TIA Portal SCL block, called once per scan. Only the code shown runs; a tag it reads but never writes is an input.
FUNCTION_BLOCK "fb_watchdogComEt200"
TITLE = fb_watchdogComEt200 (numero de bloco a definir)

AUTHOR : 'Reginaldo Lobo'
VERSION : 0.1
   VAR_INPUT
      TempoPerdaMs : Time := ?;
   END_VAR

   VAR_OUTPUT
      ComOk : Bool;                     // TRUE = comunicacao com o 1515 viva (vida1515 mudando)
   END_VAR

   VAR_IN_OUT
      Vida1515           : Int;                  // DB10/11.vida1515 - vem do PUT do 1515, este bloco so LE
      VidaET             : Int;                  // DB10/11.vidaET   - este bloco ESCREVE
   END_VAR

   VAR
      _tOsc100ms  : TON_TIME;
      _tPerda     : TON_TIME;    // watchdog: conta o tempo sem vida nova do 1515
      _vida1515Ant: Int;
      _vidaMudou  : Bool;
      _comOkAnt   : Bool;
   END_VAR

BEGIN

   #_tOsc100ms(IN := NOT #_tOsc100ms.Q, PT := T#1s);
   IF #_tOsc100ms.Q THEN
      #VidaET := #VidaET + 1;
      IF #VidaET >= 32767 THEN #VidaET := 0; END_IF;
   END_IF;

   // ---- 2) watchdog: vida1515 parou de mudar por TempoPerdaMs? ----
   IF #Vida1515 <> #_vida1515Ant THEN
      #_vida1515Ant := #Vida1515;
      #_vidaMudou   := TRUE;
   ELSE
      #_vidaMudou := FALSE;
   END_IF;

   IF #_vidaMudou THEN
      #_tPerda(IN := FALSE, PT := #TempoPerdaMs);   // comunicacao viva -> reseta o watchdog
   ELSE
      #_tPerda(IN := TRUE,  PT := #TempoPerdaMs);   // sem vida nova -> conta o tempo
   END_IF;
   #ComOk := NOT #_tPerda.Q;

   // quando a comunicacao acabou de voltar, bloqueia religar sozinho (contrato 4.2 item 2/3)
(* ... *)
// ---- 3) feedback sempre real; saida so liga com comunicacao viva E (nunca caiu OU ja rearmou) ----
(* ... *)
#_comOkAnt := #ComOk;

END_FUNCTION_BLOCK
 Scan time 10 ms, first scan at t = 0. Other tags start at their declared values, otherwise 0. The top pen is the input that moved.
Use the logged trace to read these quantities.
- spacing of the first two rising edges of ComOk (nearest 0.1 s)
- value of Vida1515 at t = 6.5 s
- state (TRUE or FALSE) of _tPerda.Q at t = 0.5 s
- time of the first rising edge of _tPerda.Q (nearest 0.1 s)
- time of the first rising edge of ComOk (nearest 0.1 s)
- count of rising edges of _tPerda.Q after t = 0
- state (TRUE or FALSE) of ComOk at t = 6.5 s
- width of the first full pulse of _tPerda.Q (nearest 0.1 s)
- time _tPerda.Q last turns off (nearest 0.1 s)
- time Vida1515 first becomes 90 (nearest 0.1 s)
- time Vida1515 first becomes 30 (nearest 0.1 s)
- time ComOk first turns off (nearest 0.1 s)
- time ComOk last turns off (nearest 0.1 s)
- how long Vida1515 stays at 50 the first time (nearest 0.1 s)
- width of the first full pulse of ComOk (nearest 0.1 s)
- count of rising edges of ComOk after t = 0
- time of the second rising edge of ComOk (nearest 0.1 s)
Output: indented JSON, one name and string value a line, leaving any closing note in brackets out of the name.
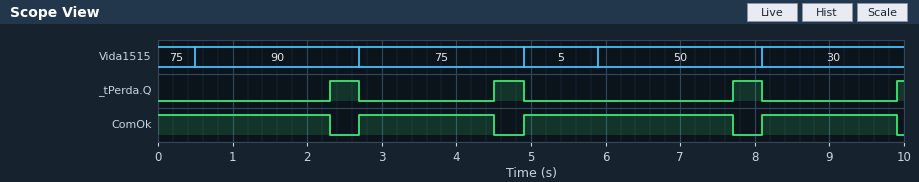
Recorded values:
{
  "spacing of the first two rising edges of ComOk": "2.2 s",
  "value of Vida1515 at t = 6.5 s": "50",
  "state (TRUE or FALSE) of _tPerda.Q at t = 0.5 s": "FALSE",
  "time of the first rising edge of _tPerda.Q": "2.3 s",
  "time of the first rising edge of ComOk": "2.7 s",
  "count of rising edges of _tPerda.Q after t = 0": "4",
  "state (TRUE or FALSE) of ComOk at t = 6.5 s": "TRUE",
  "width of the first full pulse of _tPerda.Q": "0.4 s",
  "time _tPerda.Q last turns off": "8.1 s",
  "time Vida1515 first becomes 90": "0.5 s",
  "time Vida1515 first becomes 30": "8.1 s",
  "time ComOk first turns off": "2.3 s",
  "time ComOk last turns off": "9.9 s",
  "how long Vida1515 stays at 50 the first time": "2.2 s",
  "width of the first full pulse of ComOk": "1.8 s",
  "count of rising edges of ComOk after t = 0": "3",
  "time of the second rising edge of ComOk": "4.9 s"
}
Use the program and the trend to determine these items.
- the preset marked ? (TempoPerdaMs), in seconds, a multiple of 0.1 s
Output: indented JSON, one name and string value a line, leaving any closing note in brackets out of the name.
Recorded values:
{
  "the preset marked ? (TempoPerdaMs), in seconds, a multiple of 0.1 s": "1.8 s"
}
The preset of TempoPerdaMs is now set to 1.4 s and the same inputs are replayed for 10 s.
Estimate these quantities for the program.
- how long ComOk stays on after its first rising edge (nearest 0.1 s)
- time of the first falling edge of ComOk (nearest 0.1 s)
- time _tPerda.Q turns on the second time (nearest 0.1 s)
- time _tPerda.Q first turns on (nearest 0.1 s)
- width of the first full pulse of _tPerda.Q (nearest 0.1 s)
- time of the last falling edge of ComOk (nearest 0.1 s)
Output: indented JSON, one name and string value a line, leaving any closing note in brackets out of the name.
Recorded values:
{
  "how long ComOk stays on after its first rising edge": "1.4 s",
  "time of the first falling edge of ComOk": "1.9 s",
  "time _tPerda.Q turns on the second time": "4.1 s",
  "time _tPerda.Q first turns on": "1.9 s",
  "width of the first full pulse of _tPerda.Q": "0.8 s",
  "time of the last falling edge of ComOk": "9.5 s"
}
